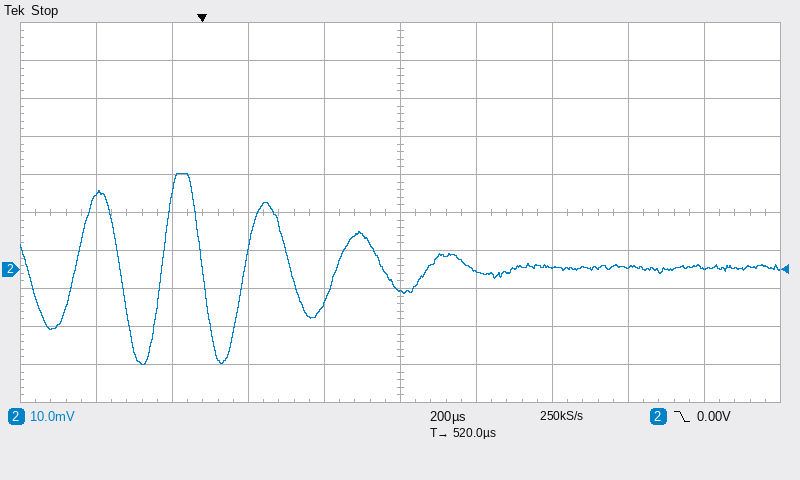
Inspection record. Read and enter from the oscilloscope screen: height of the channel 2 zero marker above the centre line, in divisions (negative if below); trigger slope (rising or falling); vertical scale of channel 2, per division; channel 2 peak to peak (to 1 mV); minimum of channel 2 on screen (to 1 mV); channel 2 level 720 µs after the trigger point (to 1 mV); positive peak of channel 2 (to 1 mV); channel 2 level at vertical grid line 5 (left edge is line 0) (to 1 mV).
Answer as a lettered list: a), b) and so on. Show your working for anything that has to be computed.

a) -1.5 div
b) falling
c) 10 mV
d) 25 mV − (-25 mV) = 50 mV
e) -25 mV
f) 0 mV
g) 25 mV
h) -6 mV
